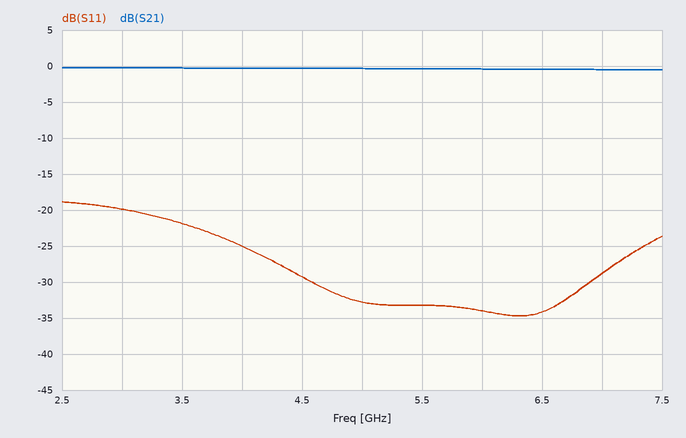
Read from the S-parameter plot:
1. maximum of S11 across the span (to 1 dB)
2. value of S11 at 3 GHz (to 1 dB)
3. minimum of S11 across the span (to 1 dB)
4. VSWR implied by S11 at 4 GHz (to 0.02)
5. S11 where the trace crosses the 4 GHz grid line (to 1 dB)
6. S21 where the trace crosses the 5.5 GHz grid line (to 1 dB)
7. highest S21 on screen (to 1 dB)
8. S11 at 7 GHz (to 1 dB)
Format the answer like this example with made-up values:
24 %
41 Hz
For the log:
-19 dB
-20 dB
-35 dB
1.12
-25 dB
0 dB
0 dB
-29 dB
